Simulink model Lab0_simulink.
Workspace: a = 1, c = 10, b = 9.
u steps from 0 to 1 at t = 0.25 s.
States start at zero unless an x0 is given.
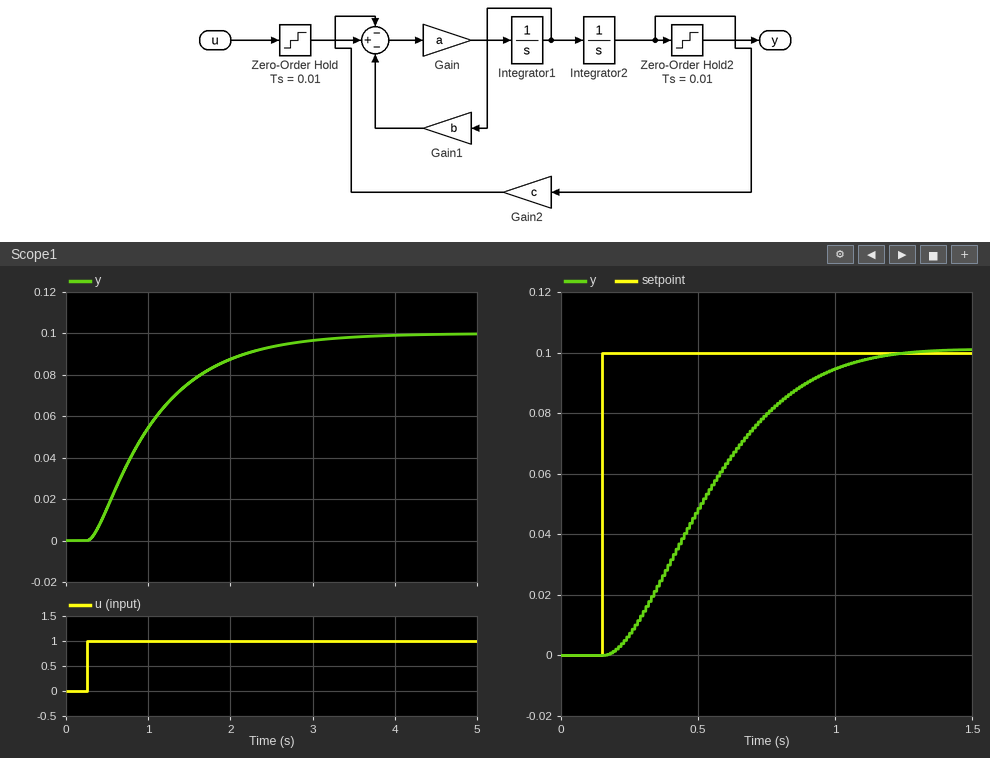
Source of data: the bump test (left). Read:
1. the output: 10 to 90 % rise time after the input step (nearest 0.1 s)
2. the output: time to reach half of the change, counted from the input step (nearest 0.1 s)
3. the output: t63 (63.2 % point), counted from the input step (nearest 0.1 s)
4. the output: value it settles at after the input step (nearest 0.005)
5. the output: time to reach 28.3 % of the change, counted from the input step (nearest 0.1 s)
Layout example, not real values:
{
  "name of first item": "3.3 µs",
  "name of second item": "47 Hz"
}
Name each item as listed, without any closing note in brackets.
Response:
{
  "the output: 10 to 90 % rise time after the input step": "1.7 s",
  "the output: time to reach half of the change, counted from the input step": "0.7 s",
  "the output: t63 (63.2 % point), counted from the input step": "0.9 s",
  "the output: value it settles at after the input step": "0.100",
  "the output: time to reach 28.3 % of the change, counted from the input step": "0.4 s"
}
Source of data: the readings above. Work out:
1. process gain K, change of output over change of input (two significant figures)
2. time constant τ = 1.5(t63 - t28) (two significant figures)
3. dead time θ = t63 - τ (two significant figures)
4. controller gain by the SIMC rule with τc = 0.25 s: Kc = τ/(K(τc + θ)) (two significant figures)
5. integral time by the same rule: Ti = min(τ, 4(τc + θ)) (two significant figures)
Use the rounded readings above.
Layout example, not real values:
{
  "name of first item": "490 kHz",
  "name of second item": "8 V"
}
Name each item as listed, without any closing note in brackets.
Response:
{
  "process gain K, change of output over change of input": "0.10",
  "time constant τ = 1.5(t63 - t28)": "0.75 s",
  "dead time θ = t63 - τ": "0.15 s",
  "controller gain by the SIMC rule with τc = 0.25 s: Kc = τ/(K(τc + θ))": "19",
  "integral time by the same rule: Ti = min(τ, 4(τc + θ))": "0.75 s"
}
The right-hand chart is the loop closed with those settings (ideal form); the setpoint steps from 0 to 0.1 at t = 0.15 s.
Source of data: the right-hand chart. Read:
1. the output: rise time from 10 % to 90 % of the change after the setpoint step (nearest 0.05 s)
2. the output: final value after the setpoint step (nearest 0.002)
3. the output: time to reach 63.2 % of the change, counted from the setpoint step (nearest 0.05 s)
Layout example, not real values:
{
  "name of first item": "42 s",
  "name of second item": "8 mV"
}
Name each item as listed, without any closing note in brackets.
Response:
{
  "the output: rise time from 10 % to 90 % of the change after the setpoint step": "0.65 s",
  "the output: final value after the setpoint step": "0.100",
  "the output: time to reach 63.2 % of the change, counted from the setpoint step": "0.45 s"
}
